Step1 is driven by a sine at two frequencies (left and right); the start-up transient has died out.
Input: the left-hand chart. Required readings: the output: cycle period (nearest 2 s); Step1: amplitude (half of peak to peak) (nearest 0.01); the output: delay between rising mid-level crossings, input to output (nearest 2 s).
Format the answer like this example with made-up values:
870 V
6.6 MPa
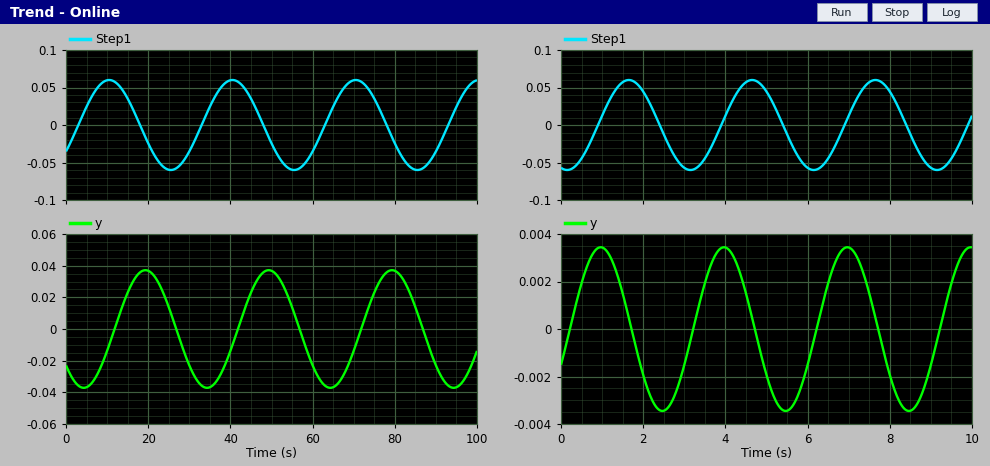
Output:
30 s
0.06
8 s
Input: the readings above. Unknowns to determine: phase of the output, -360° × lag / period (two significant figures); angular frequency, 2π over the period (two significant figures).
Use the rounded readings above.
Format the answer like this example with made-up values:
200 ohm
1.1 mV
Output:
-96°
0.21 rad/s
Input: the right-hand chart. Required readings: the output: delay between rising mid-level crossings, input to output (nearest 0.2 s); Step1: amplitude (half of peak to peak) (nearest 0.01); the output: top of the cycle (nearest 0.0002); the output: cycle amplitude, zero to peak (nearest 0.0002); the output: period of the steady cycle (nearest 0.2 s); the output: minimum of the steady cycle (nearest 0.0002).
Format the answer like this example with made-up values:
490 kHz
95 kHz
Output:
2.4 s
0.06
0.0034
0.0034
3.0 s
-0.0034
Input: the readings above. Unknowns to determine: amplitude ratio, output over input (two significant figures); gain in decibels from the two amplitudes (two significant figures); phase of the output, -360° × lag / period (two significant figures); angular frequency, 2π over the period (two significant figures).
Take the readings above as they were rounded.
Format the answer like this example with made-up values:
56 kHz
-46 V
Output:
0.057
-25 dB
-290°
2.1 rad/s
